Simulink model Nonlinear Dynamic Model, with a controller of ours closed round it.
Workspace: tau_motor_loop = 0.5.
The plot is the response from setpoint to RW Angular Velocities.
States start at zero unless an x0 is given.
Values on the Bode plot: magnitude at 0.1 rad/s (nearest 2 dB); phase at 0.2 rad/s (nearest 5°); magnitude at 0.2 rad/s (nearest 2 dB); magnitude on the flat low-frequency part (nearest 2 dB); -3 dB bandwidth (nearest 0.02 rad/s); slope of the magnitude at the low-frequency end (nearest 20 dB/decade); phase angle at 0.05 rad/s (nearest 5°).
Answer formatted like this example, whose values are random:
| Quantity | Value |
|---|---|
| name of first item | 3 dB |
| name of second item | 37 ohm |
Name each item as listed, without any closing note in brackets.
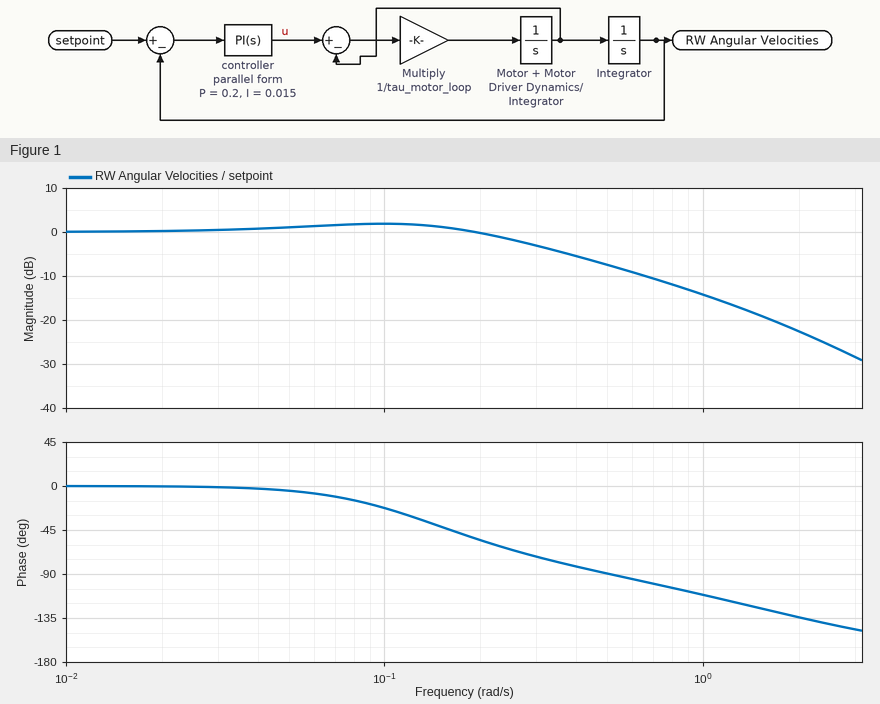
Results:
| Quantity | Value |
|---|---|
| magnitude at 0.1 rad/s | 2 dB |
| phase at 0.2 rad/s | -55° |
| magnitude at 0.2 rad/s | 0 dB |
| magnitude on the flat low-frequency part | 0 dB |
| -3 dB bandwidth | 0.30 rad/s |
| slope of the magnitude at the low-frequency end | 0 dB/decade |
| phase angle at 0.05 rad/s | -5° |
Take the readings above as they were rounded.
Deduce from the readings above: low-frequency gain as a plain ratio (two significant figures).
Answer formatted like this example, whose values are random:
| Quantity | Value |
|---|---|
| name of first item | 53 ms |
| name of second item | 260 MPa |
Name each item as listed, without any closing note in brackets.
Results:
| Quantity | Value |
|---|---|
| low-frequency gain as a plain ratio | 1.0 |
